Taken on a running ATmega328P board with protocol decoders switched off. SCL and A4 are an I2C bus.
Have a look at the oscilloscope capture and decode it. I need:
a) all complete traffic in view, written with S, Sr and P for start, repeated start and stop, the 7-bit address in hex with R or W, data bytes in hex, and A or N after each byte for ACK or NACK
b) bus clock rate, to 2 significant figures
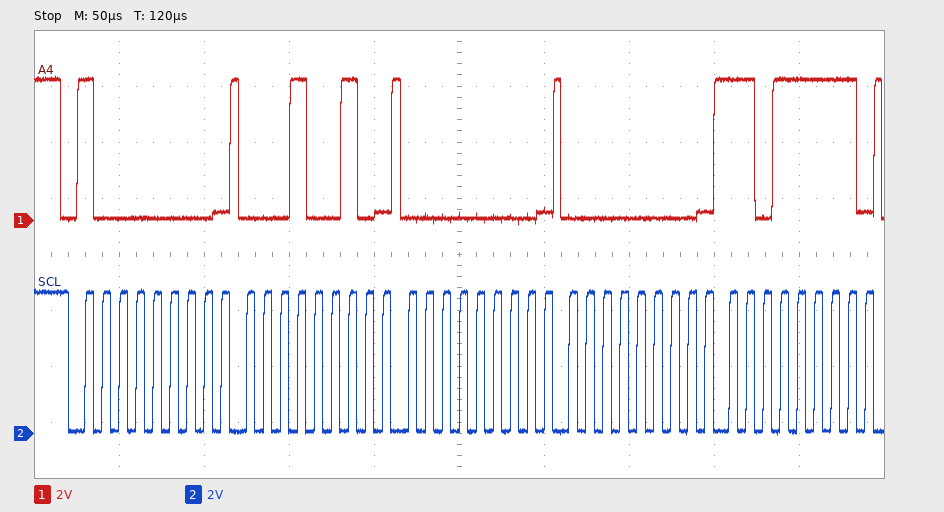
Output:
S 40W A 12 A 00 A 00 A DF A
100 kHz
